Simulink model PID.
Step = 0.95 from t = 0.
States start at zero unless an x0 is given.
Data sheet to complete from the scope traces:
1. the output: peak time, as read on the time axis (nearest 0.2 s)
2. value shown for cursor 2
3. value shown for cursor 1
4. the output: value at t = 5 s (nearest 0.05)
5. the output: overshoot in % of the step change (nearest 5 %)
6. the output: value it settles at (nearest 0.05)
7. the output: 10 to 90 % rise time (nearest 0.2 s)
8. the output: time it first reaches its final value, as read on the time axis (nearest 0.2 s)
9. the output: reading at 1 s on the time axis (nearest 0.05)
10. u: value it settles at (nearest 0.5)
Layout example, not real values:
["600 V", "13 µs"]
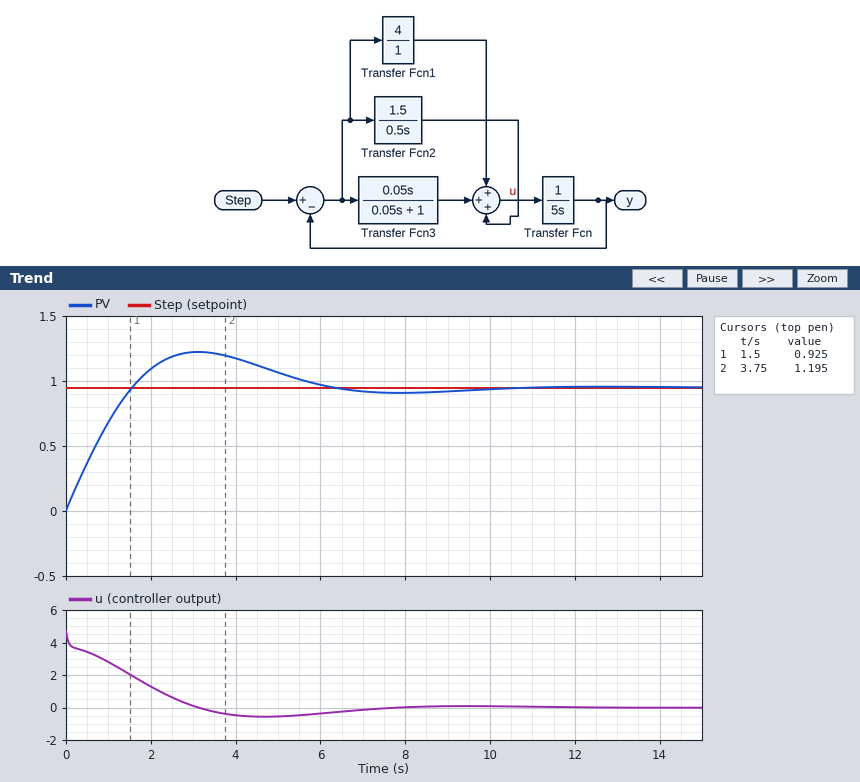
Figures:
["3.2 s", "1.195", "0.925", "1.05", "30 %", "0.95", "1.2 s", "1.6 s", "0.70", "0.0"]
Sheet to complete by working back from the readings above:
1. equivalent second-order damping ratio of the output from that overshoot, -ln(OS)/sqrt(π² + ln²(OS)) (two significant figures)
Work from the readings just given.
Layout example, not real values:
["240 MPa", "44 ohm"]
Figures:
["0.36"]
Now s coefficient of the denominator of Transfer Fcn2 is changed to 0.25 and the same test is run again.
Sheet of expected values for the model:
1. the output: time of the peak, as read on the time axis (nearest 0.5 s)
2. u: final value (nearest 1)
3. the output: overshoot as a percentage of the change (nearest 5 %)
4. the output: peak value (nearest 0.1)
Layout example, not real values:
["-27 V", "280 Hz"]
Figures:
["2.5 s", "0", "40 %", "1.3"]
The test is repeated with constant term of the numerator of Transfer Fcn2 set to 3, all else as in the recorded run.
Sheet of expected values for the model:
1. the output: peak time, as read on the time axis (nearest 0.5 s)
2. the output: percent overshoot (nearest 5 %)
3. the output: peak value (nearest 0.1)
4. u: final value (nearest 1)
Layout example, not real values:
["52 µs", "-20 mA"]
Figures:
["2.5 s", "40 %", "1.3", "0"]
